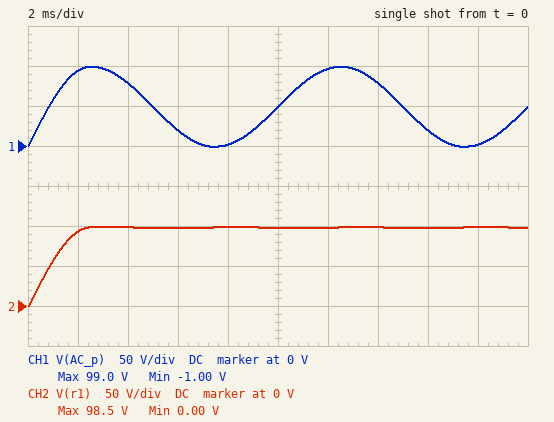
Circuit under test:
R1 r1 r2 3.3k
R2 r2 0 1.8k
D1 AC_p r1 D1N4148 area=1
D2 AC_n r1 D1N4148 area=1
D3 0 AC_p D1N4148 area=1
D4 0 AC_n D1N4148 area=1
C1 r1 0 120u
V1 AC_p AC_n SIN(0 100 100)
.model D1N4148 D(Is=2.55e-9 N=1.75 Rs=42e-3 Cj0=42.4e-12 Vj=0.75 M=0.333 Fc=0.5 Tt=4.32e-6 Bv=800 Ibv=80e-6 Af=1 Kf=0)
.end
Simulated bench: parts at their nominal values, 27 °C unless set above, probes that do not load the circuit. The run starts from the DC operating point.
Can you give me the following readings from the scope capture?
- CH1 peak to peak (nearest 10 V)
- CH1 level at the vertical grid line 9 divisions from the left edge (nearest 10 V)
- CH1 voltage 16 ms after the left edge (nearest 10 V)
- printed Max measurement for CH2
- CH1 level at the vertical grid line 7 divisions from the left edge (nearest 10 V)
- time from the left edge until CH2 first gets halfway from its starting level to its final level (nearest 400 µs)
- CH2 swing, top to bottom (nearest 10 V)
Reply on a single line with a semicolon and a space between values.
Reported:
100 V; 0 V; 20 V; 98.5 V; 80 V; 800 µs; 100 V
